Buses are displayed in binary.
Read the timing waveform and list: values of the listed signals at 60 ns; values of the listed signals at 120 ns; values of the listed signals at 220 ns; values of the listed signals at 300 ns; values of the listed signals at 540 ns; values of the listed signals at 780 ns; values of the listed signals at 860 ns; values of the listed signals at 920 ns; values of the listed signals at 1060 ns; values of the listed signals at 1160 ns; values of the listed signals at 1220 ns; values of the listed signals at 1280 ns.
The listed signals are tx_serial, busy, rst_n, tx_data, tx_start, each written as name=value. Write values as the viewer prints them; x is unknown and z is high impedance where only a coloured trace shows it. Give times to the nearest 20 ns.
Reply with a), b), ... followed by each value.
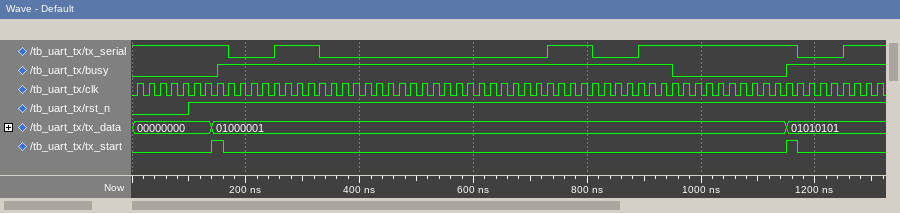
a) tx_serial=1, busy=0, rst_n=0, tx_data=00000000, tx_start=0
b) tx_serial=1, busy=0, rst_n=1, tx_data=00000000, tx_start=0
c) tx_serial=0, busy=1, rst_n=1, tx_data=01000001, tx_start=0
d) tx_serial=1, busy=1, rst_n=1, tx_data=01000001, tx_start=0
e) tx_serial=0, busy=1, rst_n=1, tx_data=01000001, tx_start=0
f) tx_serial=1, busy=1, rst_n=1, tx_data=01000001, tx_start=0
g) tx_serial=0, busy=1, rst_n=1, tx_data=01000001, tx_start=0
h) tx_serial=1, busy=1, rst_n=1, tx_data=01000001, tx_start=0
i) tx_serial=1, busy=0, rst_n=1, tx_data=01000001, tx_start=0
j) tx_serial=1, busy=1, rst_n=1, tx_data=01010101, tx_start=1
k) tx_serial=0, busy=1, rst_n=1, tx_data=01010101, tx_start=0
l) tx_serial=1, busy=1, rst_n=1, tx_data=01010101, tx_start=0
